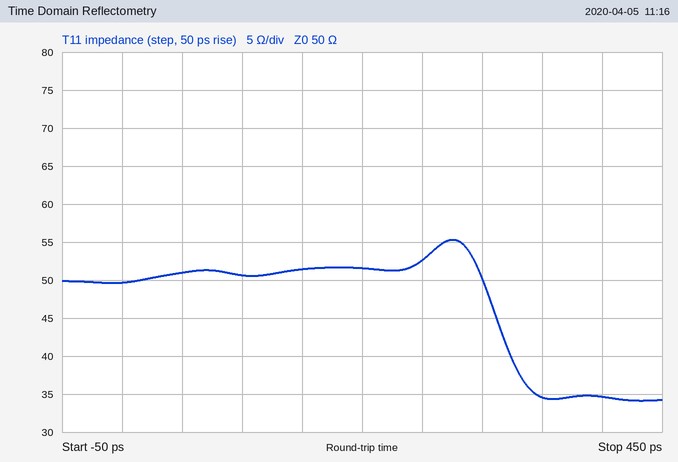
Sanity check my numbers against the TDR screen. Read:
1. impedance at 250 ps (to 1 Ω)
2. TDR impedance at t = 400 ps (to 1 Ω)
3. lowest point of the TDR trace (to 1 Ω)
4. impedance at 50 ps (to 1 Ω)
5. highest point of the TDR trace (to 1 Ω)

53 Ω
35 Ω
34 Ω
51 Ω
55 Ω
